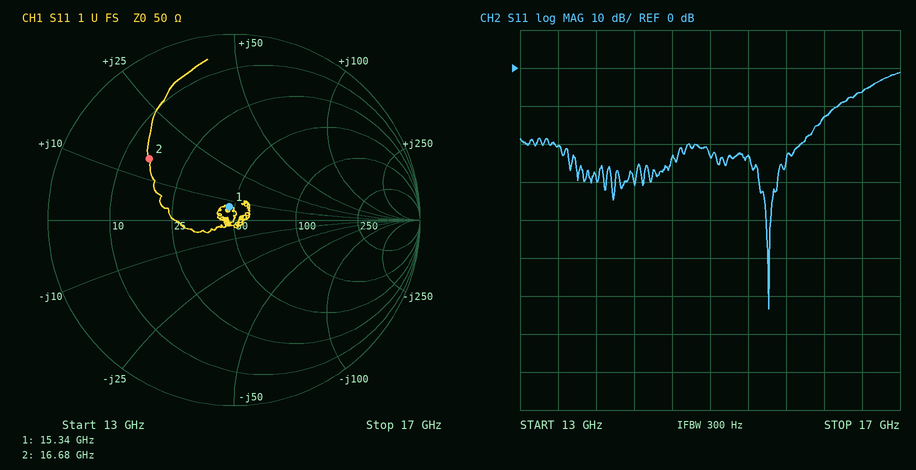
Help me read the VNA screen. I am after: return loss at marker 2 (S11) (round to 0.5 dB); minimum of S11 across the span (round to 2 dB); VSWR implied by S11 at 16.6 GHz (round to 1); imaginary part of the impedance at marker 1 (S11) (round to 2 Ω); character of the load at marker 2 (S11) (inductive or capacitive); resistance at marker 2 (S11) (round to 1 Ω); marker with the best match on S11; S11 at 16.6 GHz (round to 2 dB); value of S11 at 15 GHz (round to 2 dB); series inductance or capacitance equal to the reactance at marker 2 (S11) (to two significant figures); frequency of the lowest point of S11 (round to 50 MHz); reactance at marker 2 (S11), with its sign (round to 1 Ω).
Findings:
5.0 dB
-64 dB
3
+6 Ω
inductive
15 Ω
marker 1
-6 dB
-24 dB
140 pH
15.60 GHz
+15 Ω
